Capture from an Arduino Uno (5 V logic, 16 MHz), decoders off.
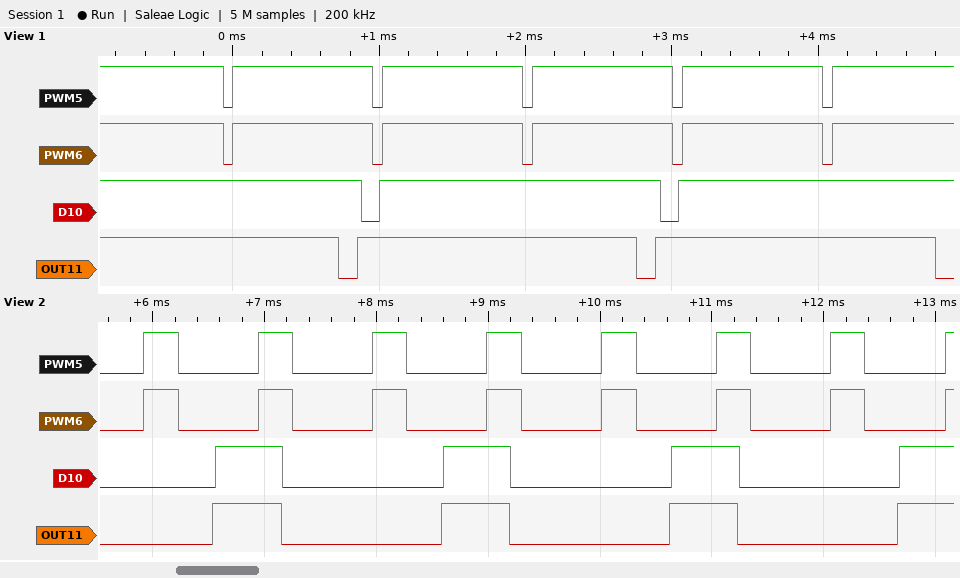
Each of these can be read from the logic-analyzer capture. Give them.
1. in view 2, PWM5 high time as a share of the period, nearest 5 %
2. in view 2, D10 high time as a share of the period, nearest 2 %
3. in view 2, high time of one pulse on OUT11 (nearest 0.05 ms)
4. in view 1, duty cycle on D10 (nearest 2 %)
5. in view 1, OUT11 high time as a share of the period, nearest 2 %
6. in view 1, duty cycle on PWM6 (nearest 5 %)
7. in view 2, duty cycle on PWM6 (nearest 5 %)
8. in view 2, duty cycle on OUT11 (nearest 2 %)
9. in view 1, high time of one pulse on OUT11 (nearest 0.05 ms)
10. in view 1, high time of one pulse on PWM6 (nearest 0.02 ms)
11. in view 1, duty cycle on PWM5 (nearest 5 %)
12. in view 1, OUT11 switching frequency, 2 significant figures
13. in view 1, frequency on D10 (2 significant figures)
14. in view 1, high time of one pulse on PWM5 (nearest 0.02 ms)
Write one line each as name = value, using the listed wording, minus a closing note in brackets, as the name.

in view 2, PWM5 high time as a share of the period, nearest 5 % = 30 %
in view 2, D10 high time as a share of the period, nearest 2 % = 30 %
in view 2, high time of one pulse on OUT11 = 0.60 ms
in view 1, duty cycle on D10 = 94 %
in view 1, OUT11 high time as a share of the period, nearest 2 % = 94 %
in view 1, duty cycle on PWM6 = 95 %
in view 2, duty cycle on PWM6 = 30 %
in view 2, duty cycle on OUT11 = 30 %
in view 1, high time of one pulse on OUT11 = 1.90 ms
in view 1, high time of one pulse on PWM6 = 0.96 ms
in view 1, duty cycle on PWM5 = 95 %
in view 1, OUT11 switching frequency, 2 significant figures = 490 Hz
in view 1, frequency on D10 = 490 Hz
in view 1, high time of one pulse on PWM5 = 0.96 ms
